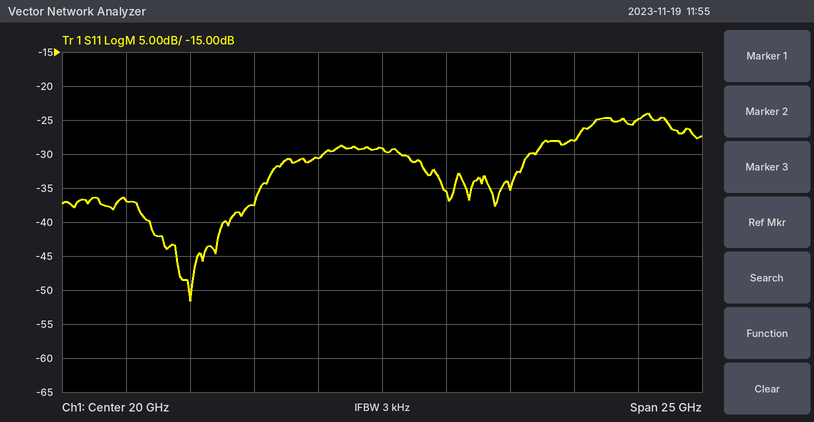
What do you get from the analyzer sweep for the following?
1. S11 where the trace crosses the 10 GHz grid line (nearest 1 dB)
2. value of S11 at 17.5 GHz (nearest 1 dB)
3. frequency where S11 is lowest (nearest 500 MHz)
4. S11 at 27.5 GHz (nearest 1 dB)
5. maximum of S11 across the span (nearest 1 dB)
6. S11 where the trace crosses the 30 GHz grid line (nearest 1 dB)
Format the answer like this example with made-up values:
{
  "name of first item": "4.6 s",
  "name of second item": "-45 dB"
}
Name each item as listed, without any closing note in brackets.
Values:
{
  "S11 where the trace crosses the 10 GHz grid line": "-37 dB",
  "value of S11 at 17.5 GHz": "-31 dB",
  "frequency where S11 is lowest": "12.5 GHz",
  "S11 at 27.5 GHz": "-28 dB",
  "maximum of S11 across the span": "-24 dB",
  "S11 where the trace crosses the 30 GHz grid line": "-25 dB"
}
